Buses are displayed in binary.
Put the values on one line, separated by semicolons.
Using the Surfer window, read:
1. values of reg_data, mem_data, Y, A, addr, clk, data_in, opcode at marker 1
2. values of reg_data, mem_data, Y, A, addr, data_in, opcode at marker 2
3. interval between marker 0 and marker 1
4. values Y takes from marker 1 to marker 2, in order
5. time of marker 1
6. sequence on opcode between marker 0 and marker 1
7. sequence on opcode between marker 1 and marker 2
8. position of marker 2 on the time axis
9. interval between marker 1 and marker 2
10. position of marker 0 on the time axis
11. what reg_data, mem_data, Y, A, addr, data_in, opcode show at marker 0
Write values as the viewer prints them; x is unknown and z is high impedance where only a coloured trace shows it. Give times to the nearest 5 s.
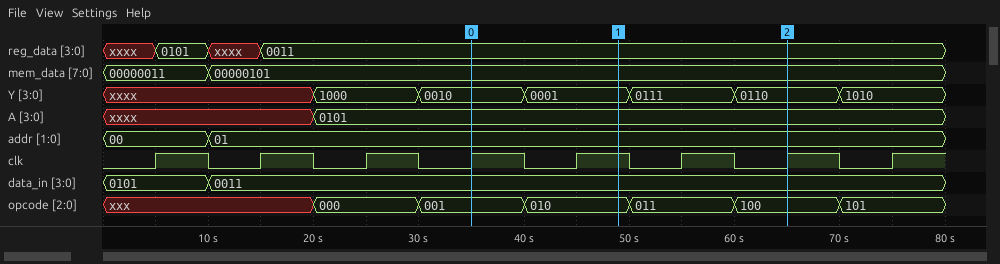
reg_data=0011, mem_data=00000101, Y=0001, A=0101, addr=01, clk=1, data_in=0011, opcode=010; reg_data=0011, mem_data=00000101, Y=0110, A=0101, addr=01, data_in=0011, opcode=100; 15 s; 0001, 0111, 0110; 50 s; 001, 010; 010, 011, 100; 65 s; 15 s; 35 s; reg_data=0011, mem_data=00000101, Y=0010, A=0101, addr=01, data_in=0011, opcode=001
